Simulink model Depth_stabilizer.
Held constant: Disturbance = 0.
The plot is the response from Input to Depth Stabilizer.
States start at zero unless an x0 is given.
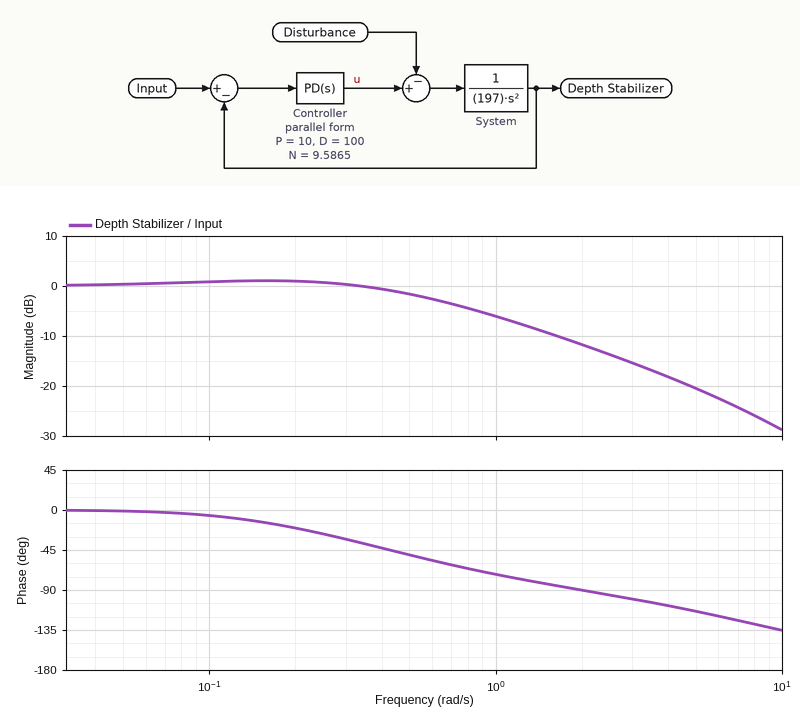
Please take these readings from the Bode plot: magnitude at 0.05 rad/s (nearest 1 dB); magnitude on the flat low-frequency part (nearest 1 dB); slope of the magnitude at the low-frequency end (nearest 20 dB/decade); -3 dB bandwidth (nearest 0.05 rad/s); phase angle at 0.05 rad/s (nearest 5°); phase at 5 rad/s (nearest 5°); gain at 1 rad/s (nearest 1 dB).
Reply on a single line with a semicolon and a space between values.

0 dB; 0 dB; 0 dB/decade; 0.60 rad/s; 0°; -115°; -6 dB
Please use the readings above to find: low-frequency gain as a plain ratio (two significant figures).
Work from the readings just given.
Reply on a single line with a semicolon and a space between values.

1.0
